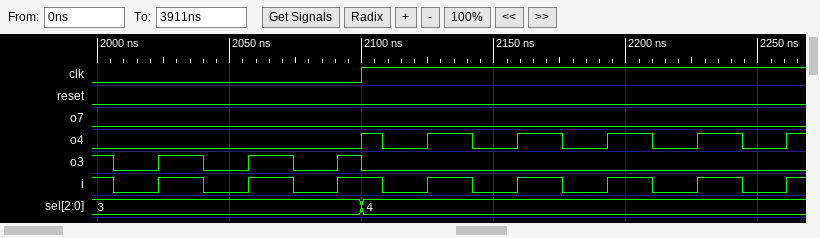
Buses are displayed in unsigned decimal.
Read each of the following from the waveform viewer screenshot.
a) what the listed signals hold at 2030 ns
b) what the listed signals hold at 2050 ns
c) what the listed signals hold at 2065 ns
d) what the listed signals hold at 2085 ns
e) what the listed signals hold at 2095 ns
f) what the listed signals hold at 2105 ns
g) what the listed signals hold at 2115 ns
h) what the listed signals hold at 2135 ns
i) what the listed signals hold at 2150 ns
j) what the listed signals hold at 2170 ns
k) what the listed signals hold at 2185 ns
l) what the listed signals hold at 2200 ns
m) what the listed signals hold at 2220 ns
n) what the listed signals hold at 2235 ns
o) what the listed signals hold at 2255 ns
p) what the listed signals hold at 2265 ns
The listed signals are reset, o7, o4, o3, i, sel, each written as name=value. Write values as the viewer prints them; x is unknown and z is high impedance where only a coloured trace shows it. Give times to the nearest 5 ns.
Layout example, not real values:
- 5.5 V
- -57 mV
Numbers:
- reset=0, o7=0, o4=0, o3=1, i=1, sel=3
- reset=0, o7=0, o4=0, o3=0, i=0, sel=3
- reset=0, o7=0, o4=0, o3=1, i=1, sel=3
- reset=0, o7=0, o4=0, o3=0, i=0, sel=3
- reset=0, o7=0, o4=0, o3=1, i=1, sel=3
- reset=0, o7=0, o4=1, o3=0, i=1, sel=4
- reset=0, o7=0, o4=0, o3=0, i=0, sel=4
- reset=0, o7=0, o4=1, o3=0, i=1, sel=4
- reset=0, o7=0, o4=0, o3=0, i=0, sel=4
- reset=0, o7=0, o4=1, o3=0, i=1, sel=4
- reset=0, o7=0, o4=0, o3=0, i=0, sel=4
- reset=0, o7=0, o4=1, o3=0, i=1, sel=4
- reset=0, o7=0, o4=0, o3=0, i=0, sel=4
- reset=0, o7=0, o4=1, o3=0, i=1, sel=4
- reset=0, o7=0, o4=0, o3=0, i=0, sel=4
- reset=0, o7=0, o4=1, o3=0, i=1, sel=4
